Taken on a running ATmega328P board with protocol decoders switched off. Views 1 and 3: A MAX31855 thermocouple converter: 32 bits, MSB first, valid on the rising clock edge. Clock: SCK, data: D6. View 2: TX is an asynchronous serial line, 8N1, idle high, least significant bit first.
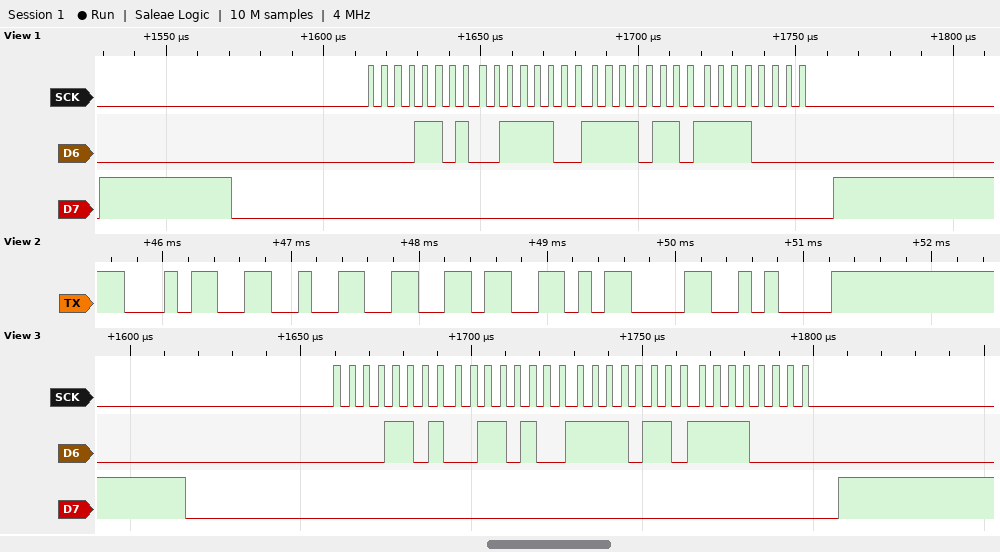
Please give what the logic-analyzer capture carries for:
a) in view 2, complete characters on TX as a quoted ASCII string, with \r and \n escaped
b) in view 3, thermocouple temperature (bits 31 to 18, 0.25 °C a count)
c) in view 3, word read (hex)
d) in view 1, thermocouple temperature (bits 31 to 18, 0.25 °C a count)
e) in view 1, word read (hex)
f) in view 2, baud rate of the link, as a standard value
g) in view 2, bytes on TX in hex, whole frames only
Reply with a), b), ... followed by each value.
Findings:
a) "426\r\n"
b) 211.25 °C
c) 0x0D34F6F0
d) 211.75 °C
e) 0x0D3CF6F0
f) 9600 baud
g) 34 32 36 0D 0A
